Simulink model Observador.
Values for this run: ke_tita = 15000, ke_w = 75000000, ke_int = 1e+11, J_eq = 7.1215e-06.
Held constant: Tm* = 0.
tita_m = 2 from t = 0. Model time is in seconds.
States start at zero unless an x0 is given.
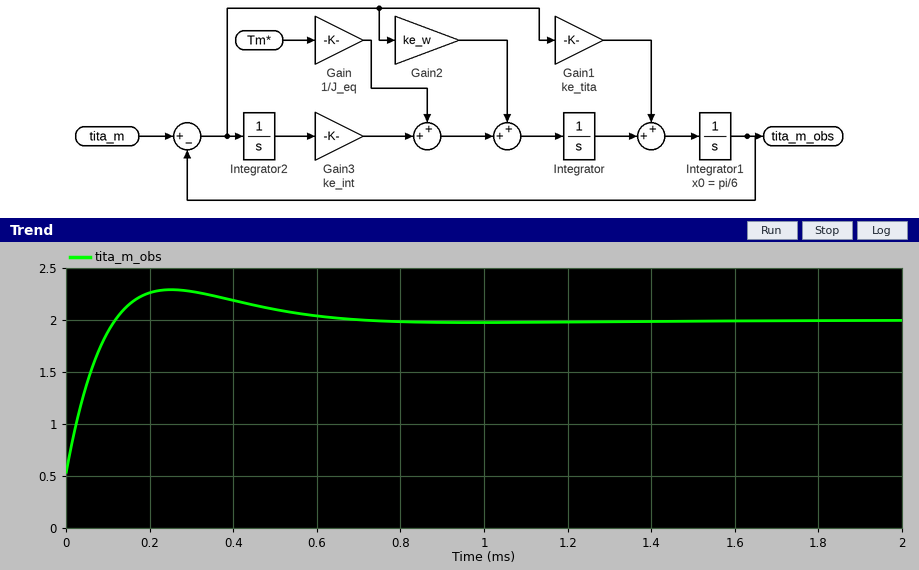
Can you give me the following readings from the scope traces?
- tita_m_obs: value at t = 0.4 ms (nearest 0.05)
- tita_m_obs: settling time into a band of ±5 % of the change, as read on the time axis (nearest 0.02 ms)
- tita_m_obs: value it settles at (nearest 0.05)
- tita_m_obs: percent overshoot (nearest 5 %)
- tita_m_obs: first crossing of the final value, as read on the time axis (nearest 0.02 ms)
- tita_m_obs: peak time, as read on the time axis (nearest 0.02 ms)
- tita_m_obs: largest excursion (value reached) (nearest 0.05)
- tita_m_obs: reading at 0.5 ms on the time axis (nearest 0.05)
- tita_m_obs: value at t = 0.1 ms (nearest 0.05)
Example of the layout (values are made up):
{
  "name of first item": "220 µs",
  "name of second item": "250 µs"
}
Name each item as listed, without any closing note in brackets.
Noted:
{
  "tita_m_obs: value at t = 0.4 ms": "2.20",
  "tita_m_obs: settling time into a band of ±5 % of the change, as read on the time axis": "0.54 ms",
  "tita_m_obs: value it settles at": "2.00",
  "tita_m_obs: percent overshoot": "20 %",
  "tita_m_obs: first crossing of the final value, as read on the time axis": "0.12 ms",
  "tita_m_obs: peak time, as read on the time axis": "0.26 ms",
  "tita_m_obs: largest excursion (value reached)": "2.30",
  "tita_m_obs: reading at 0.5 ms on the time axis": "2.10",
  "tita_m_obs: value at t = 0.1 ms": "1.90"
}
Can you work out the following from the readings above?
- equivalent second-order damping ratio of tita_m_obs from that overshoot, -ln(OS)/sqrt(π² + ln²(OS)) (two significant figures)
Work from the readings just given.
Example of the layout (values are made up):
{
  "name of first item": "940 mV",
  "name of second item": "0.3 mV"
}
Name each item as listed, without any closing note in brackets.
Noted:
{
  "equivalent second-order damping ratio of tita_m_obs from that overshoot, -ln(OS)/sqrt(π² + ln²(OS))": "0.46"
}
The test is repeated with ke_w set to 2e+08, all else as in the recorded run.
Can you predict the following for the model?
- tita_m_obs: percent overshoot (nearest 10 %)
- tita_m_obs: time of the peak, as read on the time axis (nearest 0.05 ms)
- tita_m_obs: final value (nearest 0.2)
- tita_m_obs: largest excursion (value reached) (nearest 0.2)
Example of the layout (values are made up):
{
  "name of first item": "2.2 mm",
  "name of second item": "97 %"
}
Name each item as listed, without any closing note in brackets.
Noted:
{
  "tita_m_obs: percent overshoot": "30 %",
  "tita_m_obs: time of the peak, as read on the time axis": "0.15 ms",
  "tita_m_obs: final value": "2.0",
  "tita_m_obs: largest excursion (value reached)": "2.4"
}
